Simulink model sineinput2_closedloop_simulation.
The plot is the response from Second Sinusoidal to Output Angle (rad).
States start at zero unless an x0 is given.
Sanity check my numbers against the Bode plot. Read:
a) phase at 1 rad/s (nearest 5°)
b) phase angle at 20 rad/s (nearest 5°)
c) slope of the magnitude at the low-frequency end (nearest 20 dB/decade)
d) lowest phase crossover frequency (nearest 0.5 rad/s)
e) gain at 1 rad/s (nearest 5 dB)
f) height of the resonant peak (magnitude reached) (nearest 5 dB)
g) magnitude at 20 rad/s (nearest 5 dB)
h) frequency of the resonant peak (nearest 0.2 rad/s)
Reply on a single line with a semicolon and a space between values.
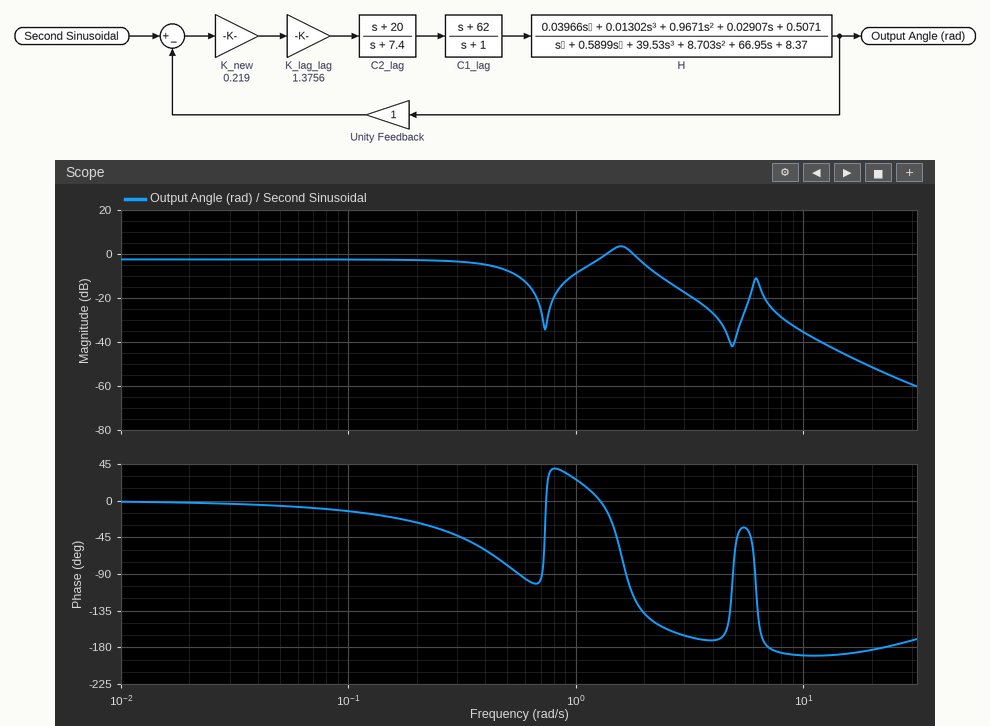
25°; -185°; 0 dB/decade; 7.0 rad/s; -10 dB; 5 dB; -50 dB; 1.6 rad/s
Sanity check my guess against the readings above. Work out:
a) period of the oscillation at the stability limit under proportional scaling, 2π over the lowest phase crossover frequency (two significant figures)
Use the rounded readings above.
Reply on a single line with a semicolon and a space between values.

0.90 s
